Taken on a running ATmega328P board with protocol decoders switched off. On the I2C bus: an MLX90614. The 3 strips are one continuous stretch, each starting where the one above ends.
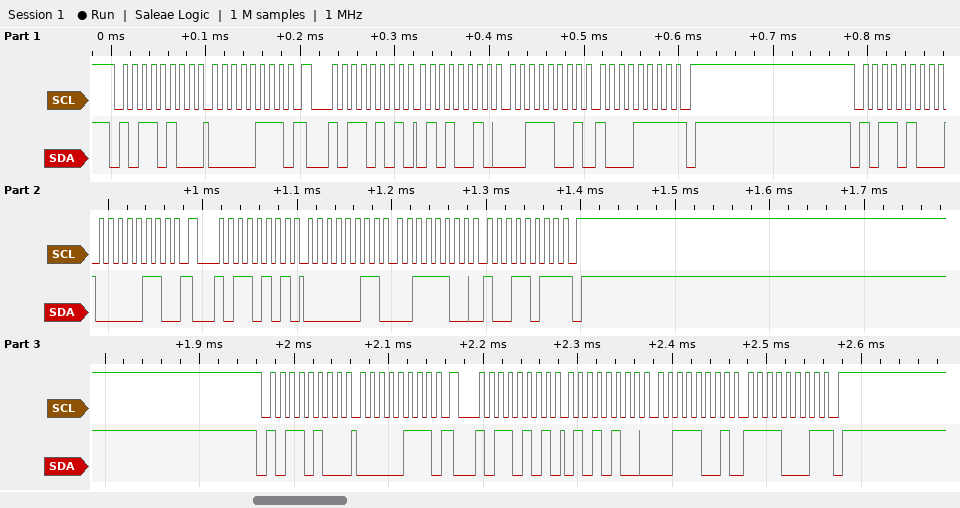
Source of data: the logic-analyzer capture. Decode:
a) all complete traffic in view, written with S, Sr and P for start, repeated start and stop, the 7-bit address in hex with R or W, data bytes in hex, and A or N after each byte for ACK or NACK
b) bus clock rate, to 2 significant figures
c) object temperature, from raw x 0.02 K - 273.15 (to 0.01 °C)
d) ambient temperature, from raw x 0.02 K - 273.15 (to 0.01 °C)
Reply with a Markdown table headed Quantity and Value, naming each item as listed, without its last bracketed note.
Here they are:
| Quantity | Value |
|---|---|
| all complete traffic in view, written with S, Sr and P for start, repeated start and stop, the 7-bit address in hex with R or W, data bytes in hex, and A or N after each byte for ACK or NACK | S 5AW A 07 A Sr 5AR A 52 A 39 A 8F N P S 5AW A 06 A Sr 5AR A 03 A 3C A 9B N P S 5AW A 07 A Sr 5AR A 54 A 39 A F1 N P |
| bus clock rate, to 2 significant figures | 100 kHz |
| object temperature, from raw x 0.02 K - 273.15 | 20.33 °C |
| ambient temperature, from raw x 0.02 K - 273.15 | 34.11 °C |
